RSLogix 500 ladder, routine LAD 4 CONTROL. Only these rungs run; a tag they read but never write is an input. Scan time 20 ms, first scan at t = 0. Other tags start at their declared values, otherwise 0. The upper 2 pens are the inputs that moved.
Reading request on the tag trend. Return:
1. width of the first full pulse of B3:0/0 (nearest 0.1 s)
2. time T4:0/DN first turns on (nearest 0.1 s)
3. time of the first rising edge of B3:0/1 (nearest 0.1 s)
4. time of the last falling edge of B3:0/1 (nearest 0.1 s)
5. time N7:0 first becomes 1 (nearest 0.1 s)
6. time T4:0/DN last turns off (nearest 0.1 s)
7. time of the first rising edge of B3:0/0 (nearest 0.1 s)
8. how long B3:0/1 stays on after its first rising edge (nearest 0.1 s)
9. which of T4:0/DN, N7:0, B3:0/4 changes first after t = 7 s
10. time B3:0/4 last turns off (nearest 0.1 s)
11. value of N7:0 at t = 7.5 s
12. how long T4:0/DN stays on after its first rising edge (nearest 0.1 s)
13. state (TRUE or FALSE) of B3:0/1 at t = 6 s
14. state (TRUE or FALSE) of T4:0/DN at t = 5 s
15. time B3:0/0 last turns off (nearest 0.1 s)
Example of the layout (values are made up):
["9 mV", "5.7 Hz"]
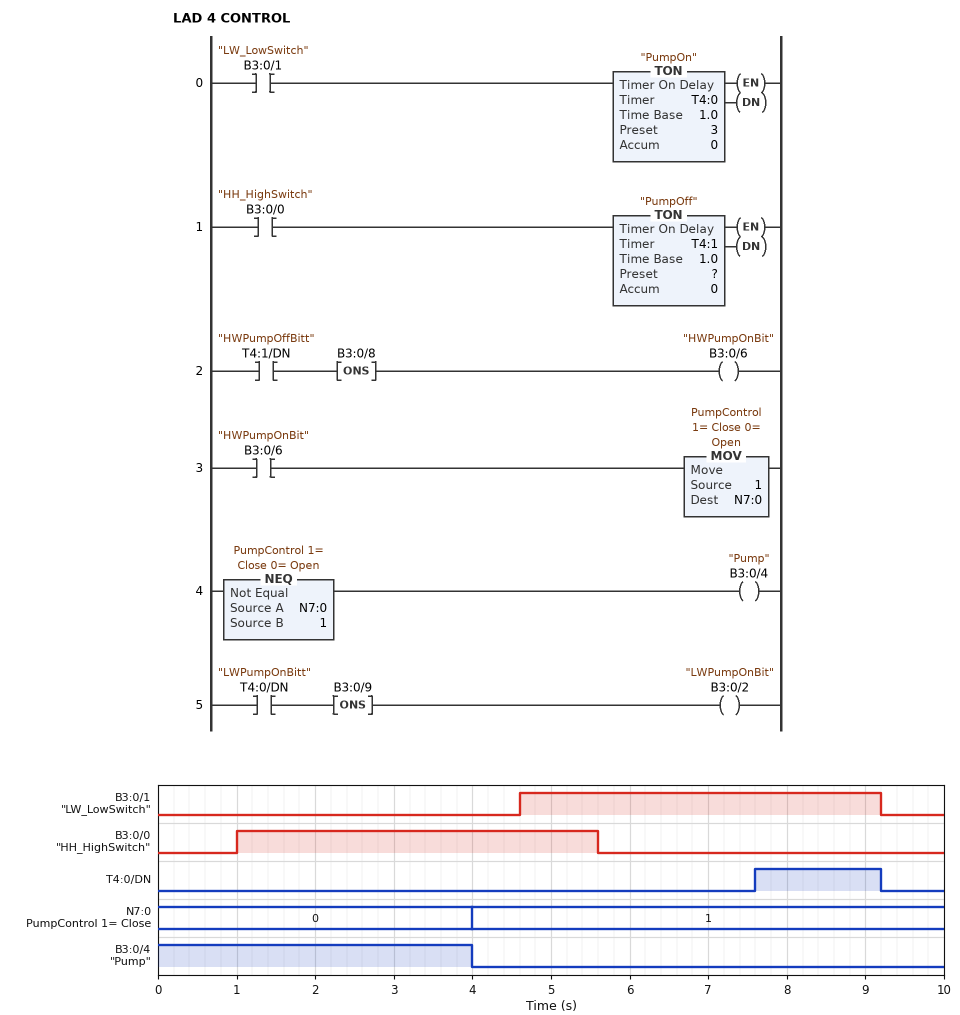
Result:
["4.6 s", "7.6 s", "4.6 s", "9.2 s", "4.0 s", "9.2 s", "1.0 s", "4.6 s", "T4:0/DN", "4.0 s", "1", "1.6 s", "TRUE", "FALSE", "5.6 s"]
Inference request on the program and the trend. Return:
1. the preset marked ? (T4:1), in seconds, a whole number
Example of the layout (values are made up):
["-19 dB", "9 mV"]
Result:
["3 s"]
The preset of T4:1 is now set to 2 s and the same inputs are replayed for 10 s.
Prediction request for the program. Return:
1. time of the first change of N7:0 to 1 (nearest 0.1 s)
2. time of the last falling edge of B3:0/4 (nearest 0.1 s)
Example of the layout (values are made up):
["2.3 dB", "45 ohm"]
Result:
["3.0 s", "3.0 s"]
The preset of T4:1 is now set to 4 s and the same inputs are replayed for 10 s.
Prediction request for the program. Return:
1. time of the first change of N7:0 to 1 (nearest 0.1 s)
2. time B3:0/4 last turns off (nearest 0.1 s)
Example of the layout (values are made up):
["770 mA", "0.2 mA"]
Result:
["5.0 s", "5.0 s"]
